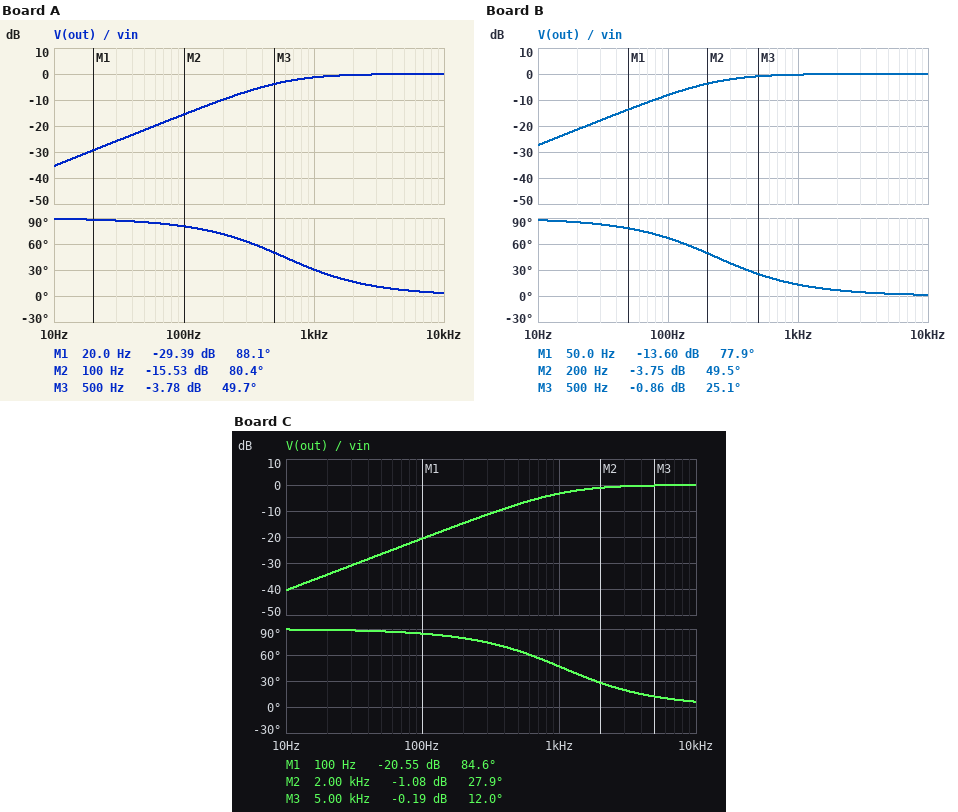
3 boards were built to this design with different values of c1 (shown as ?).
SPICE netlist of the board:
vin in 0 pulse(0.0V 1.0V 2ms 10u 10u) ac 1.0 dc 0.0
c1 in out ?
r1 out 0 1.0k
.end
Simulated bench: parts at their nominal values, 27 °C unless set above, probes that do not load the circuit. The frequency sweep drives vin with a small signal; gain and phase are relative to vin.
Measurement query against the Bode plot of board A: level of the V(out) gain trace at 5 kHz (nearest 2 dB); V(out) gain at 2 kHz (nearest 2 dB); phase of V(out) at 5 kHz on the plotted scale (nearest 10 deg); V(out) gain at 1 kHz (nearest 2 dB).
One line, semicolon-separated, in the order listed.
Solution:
0 dB; 0 dB; 10 deg; -2 dB
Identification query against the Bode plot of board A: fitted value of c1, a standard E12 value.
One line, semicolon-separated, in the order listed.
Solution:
270 nF
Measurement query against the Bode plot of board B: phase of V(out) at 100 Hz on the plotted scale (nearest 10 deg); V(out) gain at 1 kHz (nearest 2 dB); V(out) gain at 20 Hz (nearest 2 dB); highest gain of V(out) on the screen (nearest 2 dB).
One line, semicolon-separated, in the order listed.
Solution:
70 deg; 0 dB; -22 dB; 0 dB
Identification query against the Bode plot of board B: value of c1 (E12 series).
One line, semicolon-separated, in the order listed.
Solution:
680 nF
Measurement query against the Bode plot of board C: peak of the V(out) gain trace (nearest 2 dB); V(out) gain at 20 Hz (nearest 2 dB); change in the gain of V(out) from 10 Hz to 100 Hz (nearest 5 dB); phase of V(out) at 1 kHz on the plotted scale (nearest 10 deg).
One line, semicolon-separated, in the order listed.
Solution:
0 dB; -34 dB; 20 dB; 50 deg
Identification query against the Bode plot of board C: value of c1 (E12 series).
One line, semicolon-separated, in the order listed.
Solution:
150 nF
